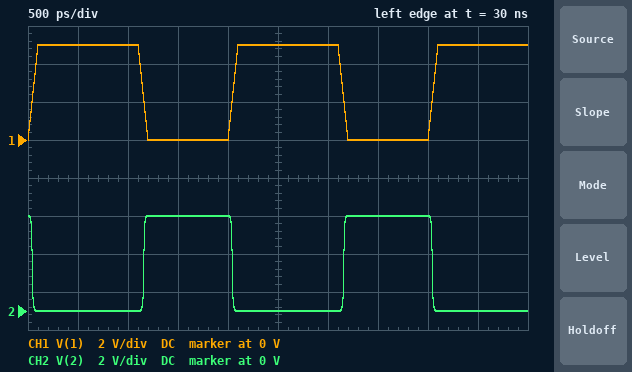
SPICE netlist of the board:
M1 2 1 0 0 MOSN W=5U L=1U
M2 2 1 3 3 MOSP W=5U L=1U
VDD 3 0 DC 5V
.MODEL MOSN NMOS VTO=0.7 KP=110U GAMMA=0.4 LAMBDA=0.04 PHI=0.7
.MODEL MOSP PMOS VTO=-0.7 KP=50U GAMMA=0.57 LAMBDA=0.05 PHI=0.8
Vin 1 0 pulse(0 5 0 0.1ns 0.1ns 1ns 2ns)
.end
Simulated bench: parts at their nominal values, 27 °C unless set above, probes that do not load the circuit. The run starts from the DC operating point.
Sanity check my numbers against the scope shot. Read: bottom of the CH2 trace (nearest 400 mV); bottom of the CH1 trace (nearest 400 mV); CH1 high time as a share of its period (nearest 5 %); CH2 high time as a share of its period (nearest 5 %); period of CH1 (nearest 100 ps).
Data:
0 V
0 V
55 %
45 %
2.0 ns
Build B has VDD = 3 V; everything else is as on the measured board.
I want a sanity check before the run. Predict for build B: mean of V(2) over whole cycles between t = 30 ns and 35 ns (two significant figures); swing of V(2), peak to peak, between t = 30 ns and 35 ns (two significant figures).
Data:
1.3 V
3.0 V
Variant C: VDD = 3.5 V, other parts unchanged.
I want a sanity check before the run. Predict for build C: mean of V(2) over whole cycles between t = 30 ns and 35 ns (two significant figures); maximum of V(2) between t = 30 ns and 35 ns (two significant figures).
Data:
1.5 V
3.5 V
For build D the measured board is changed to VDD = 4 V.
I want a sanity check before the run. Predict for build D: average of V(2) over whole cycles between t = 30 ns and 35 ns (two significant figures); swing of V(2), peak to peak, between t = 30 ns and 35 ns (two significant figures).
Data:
1.7 V
4.0 V
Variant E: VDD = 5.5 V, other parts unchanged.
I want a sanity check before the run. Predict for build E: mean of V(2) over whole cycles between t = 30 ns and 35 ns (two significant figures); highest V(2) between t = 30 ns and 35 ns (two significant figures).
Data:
2.5 V
5.5 V
